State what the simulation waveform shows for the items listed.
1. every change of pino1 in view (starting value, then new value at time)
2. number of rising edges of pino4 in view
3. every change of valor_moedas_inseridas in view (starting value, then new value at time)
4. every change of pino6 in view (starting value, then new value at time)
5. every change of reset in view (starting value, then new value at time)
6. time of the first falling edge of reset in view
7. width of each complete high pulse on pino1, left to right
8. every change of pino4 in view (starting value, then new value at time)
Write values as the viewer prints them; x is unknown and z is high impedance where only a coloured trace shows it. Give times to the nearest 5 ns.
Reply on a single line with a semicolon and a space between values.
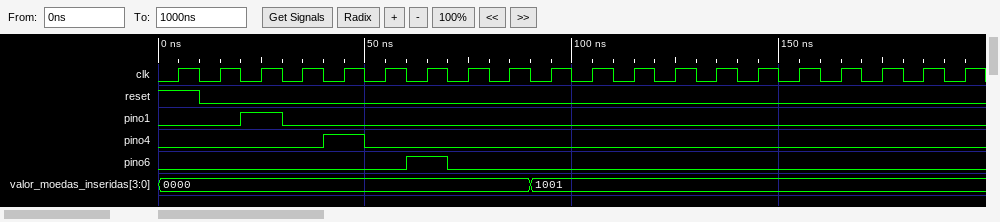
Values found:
0, 1 at 20 ns, 0 at 30 ns; 1; 0000, 1001 at 90 ns; 0, 1 at 60 ns, 0 at 70 ns; 1, 0 at 10 ns; 10 ns; 10 ns; 0, 1 at 40 ns, 0 at 50 ns
